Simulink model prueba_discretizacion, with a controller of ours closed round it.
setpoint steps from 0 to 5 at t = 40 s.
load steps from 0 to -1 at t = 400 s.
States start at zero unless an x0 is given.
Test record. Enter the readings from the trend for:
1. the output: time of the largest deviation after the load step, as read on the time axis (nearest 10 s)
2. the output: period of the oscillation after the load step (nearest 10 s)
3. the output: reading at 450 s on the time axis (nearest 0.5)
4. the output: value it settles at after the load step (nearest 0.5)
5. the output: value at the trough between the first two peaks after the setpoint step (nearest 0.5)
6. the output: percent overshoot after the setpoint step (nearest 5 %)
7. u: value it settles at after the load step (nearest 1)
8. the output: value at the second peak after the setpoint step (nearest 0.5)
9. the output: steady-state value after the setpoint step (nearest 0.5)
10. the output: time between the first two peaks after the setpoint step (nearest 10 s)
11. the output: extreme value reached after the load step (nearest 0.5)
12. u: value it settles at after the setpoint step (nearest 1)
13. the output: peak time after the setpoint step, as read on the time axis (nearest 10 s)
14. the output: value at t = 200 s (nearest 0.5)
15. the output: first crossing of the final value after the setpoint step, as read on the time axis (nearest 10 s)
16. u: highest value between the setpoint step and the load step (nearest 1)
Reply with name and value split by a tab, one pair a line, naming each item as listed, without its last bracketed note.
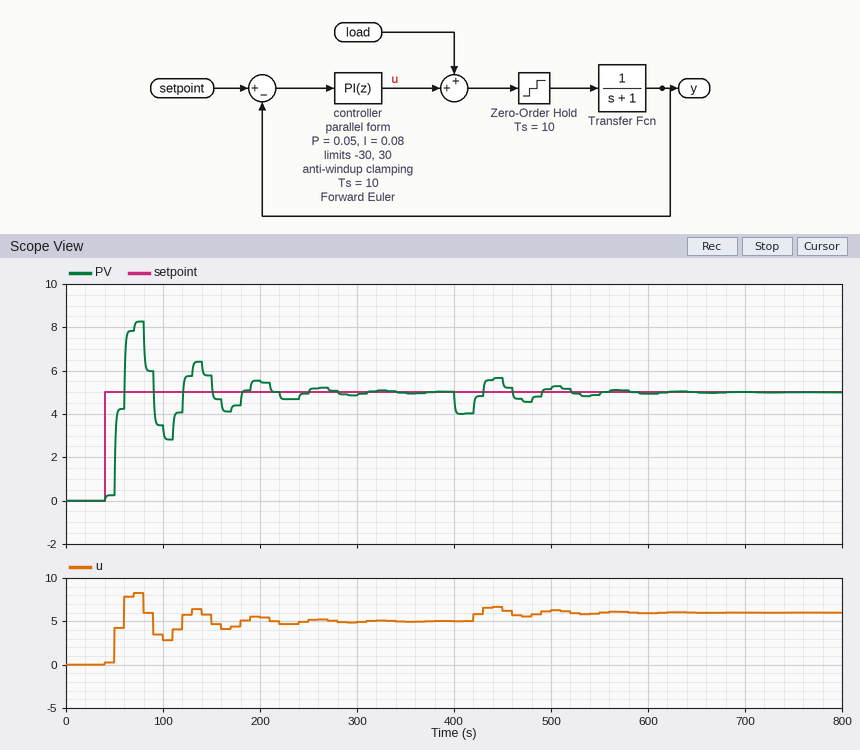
the output: time of the largest deviation after the load step, as read on the time axis	410 s
the output: period of the oscillation after the load step	70 s
the output: reading at 450 s on the time axis	5.5
the output: value it settles at after the load step	5.0
the output: value at the trough between the first two peaks after the setpoint step	3.0
the output: percent overshoot after the setpoint step	65 %
u: value it settles at after the load step	6
the output: value at the second peak after the setpoint step	6.5
the output: steady-state value after the setpoint step	5.0
the output: time between the first two peaks after the setpoint step	60 s
the output: extreme value reached after the load step	4.0
u: value it settles at after the setpoint step	5
the output: peak time after the setpoint step, as read on the time axis	80 s
the output: value at t = 200 s	5.5
the output: first crossing of the final value after the setpoint step, as read on the time axis	60 s
u: highest value between the setpoint step and the load step	8
